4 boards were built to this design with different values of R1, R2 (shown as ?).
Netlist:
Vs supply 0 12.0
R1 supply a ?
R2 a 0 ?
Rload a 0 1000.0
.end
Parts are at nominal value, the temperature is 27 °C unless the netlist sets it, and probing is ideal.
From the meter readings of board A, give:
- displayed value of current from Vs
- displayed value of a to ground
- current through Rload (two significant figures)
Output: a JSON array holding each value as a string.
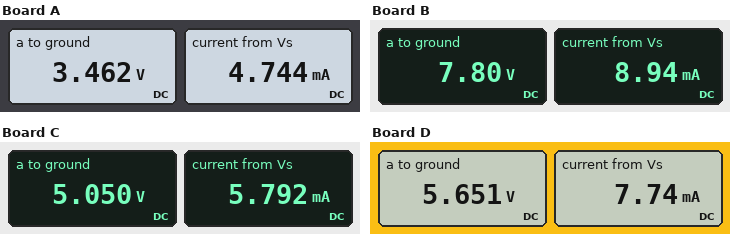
["4.744 mA", "3.462 V", "3.5 mA"]
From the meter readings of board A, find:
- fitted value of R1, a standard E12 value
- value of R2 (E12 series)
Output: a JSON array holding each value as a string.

["1.8 kΩ", "2.7 kΩ"]
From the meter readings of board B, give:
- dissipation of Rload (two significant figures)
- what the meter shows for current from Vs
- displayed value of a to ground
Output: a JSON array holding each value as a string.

["61 mW", "8.94 mA", "7.80 V"]
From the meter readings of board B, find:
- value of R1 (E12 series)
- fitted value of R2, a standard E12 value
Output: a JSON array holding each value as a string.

["470 Ω", "6.8 kΩ"]
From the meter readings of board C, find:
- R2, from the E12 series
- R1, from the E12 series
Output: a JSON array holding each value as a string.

["6.8 kΩ", "1.2 kΩ"]
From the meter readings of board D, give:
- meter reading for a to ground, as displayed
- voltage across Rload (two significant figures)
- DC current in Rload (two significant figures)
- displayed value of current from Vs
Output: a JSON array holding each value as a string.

["5.651 V", "5.7 V", "5.7 mA", "7.74 mA"]
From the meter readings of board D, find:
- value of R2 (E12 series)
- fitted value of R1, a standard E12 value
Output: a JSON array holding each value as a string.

["2.7 kΩ", "820 Ω"]
